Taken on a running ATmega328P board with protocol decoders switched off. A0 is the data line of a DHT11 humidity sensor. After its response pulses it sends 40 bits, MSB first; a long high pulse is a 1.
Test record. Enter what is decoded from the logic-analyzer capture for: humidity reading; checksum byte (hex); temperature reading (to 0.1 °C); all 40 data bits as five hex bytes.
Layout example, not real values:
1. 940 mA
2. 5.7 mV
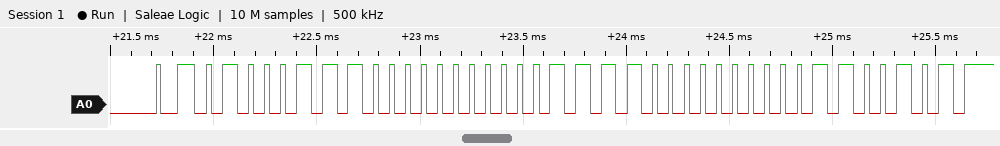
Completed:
1. 71 %
2. 0x65
3. 30.0 °C
4. 47 00 1E 00 65
